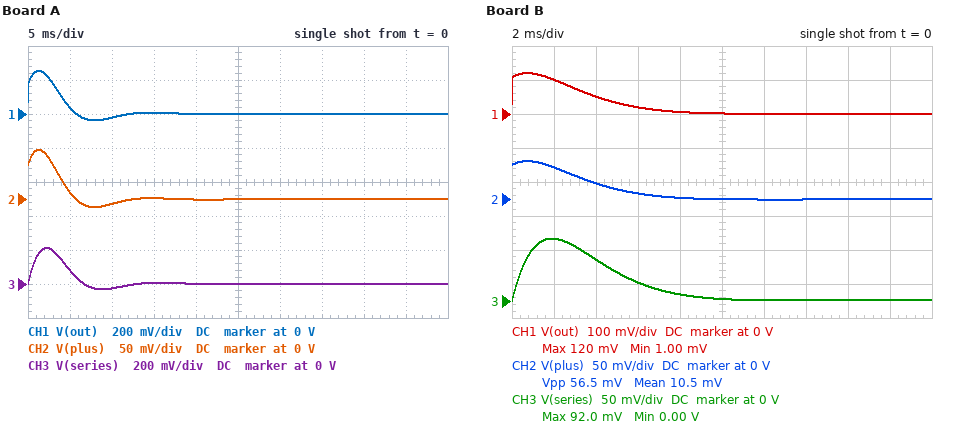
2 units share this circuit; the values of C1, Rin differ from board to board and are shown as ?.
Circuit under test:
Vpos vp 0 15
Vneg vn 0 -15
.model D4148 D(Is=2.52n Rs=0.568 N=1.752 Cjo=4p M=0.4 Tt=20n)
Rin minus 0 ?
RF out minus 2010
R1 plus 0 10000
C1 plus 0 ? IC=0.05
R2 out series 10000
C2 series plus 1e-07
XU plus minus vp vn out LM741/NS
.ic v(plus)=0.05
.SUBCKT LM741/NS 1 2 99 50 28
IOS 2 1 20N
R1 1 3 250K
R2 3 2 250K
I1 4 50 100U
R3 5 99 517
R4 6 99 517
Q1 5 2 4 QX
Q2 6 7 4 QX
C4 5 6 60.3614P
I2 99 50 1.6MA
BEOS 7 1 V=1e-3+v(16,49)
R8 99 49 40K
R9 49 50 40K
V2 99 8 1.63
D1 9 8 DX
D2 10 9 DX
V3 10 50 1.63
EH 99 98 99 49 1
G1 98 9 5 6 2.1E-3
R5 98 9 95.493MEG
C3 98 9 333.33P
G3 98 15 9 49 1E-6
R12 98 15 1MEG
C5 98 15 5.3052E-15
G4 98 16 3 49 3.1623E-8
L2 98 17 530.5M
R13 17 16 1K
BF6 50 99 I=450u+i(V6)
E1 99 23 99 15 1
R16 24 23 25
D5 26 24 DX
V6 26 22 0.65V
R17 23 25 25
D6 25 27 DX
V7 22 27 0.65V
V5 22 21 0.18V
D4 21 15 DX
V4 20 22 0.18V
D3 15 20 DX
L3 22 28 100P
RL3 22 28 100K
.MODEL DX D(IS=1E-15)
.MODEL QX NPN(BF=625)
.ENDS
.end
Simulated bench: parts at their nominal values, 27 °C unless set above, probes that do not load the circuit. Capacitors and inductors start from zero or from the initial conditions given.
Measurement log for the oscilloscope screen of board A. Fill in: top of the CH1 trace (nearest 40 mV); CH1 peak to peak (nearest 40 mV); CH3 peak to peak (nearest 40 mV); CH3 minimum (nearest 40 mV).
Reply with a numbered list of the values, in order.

1. 240 mV
2. 280 mV
3. 240 mV
4. -40 mV
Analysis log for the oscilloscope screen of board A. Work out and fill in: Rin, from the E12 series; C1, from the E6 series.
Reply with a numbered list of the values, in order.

1. 820 Ω
2. 330 nF
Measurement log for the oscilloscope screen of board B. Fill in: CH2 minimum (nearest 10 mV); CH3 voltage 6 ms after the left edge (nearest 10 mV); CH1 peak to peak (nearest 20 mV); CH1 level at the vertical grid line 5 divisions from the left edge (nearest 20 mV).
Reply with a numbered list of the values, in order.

1. 0 V
2. 30 mV
3. 120 mV
4. 0 V
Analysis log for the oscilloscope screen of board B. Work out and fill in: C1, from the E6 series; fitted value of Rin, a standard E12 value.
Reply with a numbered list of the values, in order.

1. 330 nF
2. 1.8 kΩ
